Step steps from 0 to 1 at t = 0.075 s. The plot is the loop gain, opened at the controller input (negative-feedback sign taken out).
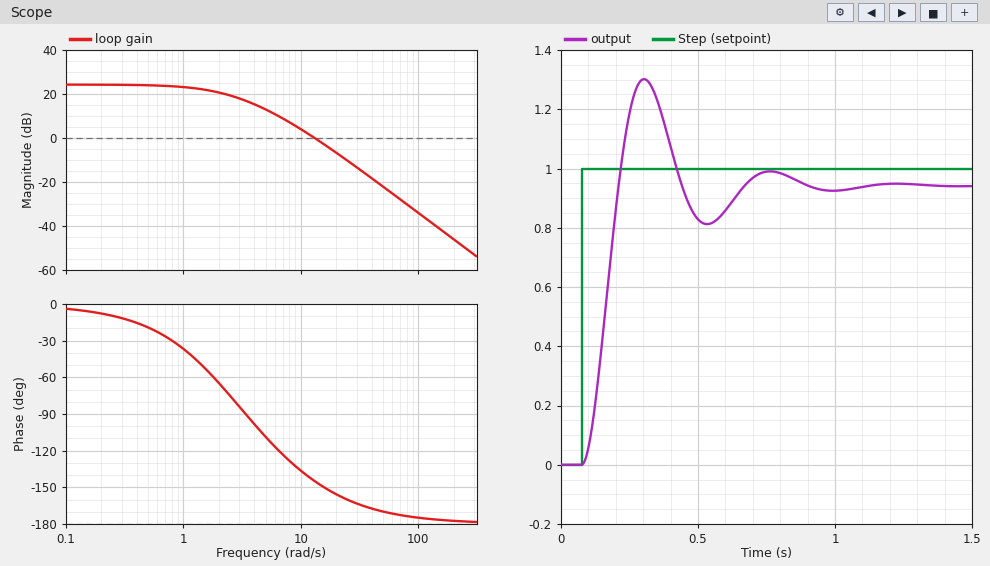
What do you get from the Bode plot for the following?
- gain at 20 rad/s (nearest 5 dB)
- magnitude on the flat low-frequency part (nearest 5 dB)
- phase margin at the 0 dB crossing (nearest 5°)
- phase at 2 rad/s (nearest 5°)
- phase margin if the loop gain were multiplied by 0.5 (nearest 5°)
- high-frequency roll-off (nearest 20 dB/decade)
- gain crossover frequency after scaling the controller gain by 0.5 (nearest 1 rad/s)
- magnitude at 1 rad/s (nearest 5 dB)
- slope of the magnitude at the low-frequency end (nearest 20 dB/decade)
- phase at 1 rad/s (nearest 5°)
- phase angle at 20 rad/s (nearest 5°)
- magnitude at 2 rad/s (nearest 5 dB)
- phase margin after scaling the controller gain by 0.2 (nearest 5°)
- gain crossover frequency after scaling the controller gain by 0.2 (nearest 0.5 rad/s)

-5 dB
25 dB
35°
-65°
50°
-40 dB/decade
9 rad/s
25 dB
0 dB/decade
-35°
-155°
20 dB
75°
4.5 rad/s
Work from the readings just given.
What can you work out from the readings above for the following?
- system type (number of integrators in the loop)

0
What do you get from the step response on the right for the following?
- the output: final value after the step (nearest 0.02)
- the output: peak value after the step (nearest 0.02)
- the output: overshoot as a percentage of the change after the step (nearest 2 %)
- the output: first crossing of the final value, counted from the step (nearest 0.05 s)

0.94
1.30
38 %
0.15 s
